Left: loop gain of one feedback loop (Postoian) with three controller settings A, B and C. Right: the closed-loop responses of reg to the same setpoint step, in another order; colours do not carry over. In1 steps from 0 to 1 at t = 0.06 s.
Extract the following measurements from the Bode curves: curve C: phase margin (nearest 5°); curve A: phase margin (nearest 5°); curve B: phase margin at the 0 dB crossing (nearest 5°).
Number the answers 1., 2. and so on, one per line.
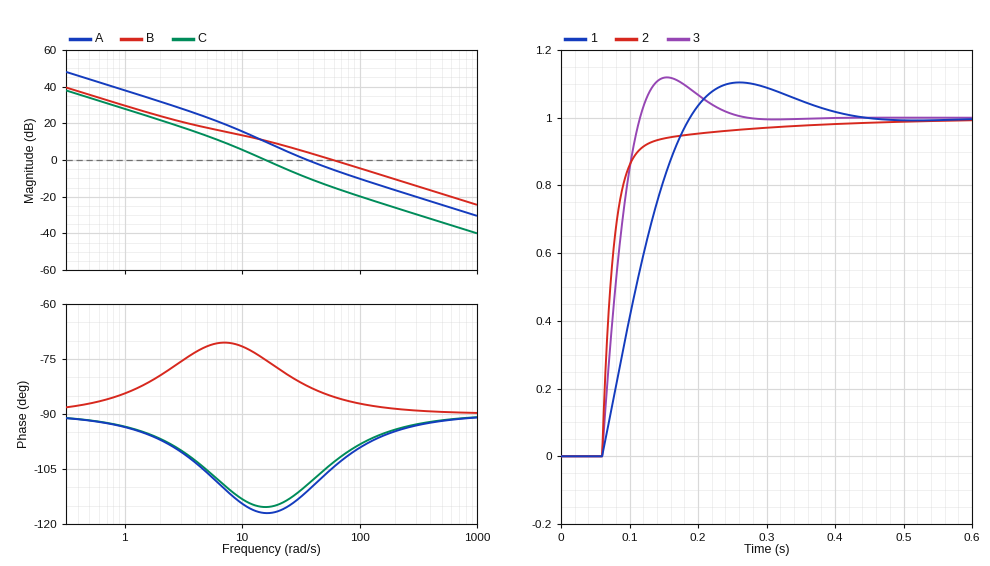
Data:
1. 65°
2. 70°
3. 95°
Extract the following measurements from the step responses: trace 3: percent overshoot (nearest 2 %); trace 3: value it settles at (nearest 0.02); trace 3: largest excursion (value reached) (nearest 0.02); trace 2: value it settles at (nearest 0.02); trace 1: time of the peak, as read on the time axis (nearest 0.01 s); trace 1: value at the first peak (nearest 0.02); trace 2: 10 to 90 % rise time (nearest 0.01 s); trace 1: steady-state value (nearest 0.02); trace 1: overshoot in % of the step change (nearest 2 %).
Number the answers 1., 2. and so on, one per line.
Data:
1. 12 %
2. 1.00
3. 1.12
4. 1.00
5. 0.26 s
6. 1.10
7. 0.05 s
8. 1.00
9. 10 %
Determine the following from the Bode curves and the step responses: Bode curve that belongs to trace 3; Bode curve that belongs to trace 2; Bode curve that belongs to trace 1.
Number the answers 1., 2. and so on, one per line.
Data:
1. A
2. B
3. C
